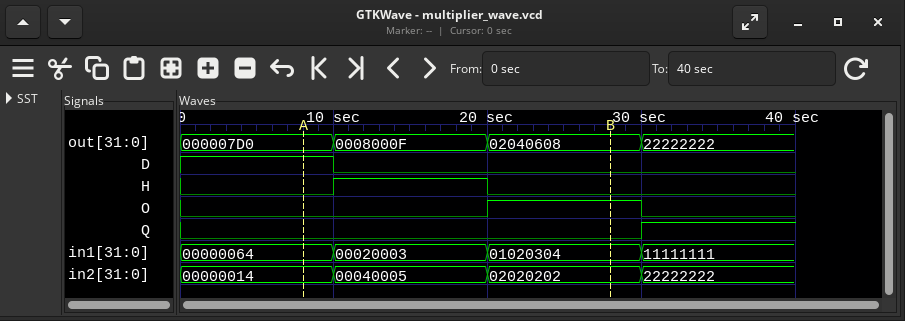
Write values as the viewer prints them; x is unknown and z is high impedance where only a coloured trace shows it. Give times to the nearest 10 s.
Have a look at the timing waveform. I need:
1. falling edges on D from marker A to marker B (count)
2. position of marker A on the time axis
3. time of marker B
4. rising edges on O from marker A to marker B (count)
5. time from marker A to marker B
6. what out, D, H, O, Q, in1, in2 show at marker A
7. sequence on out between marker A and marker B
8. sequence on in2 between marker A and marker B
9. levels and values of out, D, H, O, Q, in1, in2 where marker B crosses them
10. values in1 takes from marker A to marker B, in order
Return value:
1
10 s
30 s
1
20 s
out=000007D0, D=1, H=0, O=0, Q=0, in1=00000064, in2=00000014
000007D0, 0008000F, 02040608
00000014, 00040005, 02020202
out=02040608, D=0, H=0, O=1, Q=0, in1=01020304, in2=02020202
00000064, 00020003, 01020304
